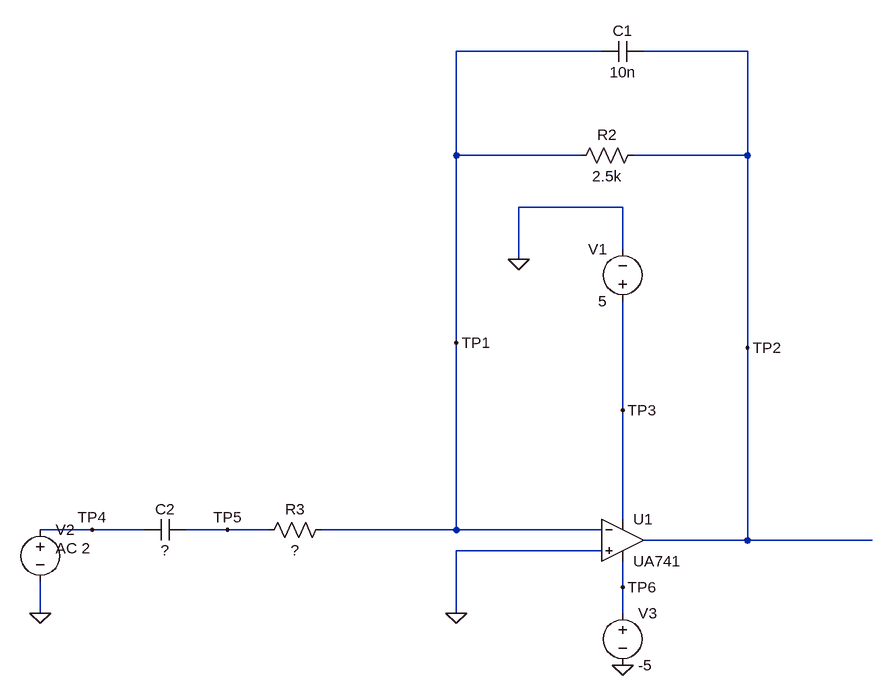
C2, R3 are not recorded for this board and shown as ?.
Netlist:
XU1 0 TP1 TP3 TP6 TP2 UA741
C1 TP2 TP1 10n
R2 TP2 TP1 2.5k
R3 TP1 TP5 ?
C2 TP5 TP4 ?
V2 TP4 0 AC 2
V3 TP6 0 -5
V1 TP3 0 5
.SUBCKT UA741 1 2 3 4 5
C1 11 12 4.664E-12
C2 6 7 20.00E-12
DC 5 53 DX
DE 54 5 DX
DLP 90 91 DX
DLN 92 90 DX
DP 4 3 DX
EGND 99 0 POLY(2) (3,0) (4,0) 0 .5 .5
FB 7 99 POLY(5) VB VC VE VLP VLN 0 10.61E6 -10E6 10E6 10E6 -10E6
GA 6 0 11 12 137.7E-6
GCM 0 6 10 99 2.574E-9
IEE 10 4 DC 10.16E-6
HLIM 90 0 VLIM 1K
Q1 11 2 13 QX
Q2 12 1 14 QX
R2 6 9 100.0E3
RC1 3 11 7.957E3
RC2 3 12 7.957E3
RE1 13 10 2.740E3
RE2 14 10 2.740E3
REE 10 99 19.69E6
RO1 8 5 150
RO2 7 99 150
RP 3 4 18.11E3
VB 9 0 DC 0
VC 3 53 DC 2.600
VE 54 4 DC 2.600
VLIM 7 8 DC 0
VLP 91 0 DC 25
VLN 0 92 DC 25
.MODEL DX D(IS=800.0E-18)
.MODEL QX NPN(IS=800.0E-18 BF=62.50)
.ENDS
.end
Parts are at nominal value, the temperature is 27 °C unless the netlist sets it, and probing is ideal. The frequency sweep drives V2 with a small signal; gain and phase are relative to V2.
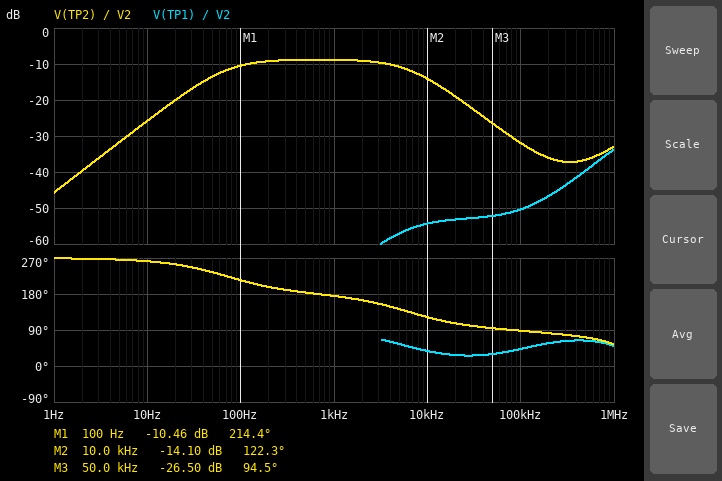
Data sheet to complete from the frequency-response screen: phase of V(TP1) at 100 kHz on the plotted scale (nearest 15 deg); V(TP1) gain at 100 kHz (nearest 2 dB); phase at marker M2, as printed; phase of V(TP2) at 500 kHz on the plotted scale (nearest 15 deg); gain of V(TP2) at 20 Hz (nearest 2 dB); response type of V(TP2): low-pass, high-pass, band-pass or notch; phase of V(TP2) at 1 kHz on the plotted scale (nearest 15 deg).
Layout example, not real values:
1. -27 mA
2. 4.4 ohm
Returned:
1. 45 deg
2. -50 dB
3. 122.3 deg
4. 75 deg
5. -20 dB
6. band-pass
7. 180 deg
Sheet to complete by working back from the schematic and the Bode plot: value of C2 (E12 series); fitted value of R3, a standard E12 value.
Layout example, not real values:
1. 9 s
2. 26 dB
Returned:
1. 330 nF
2. 6.8 kΩ
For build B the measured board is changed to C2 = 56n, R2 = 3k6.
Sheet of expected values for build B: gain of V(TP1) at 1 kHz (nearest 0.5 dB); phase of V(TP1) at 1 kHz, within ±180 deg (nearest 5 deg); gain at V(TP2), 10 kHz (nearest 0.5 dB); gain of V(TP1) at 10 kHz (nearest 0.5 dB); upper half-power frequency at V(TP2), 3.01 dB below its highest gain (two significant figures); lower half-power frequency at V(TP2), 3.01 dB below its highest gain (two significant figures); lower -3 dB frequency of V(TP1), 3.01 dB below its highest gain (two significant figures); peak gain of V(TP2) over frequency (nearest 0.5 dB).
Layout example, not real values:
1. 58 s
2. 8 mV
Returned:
1. -67.0 dB
2. 100 deg
3. -13.5 dB
4. -54.0 dB
5. 5.2 kHz
6. 360 Hz
7. 940 kHz
8. -6.5 dB
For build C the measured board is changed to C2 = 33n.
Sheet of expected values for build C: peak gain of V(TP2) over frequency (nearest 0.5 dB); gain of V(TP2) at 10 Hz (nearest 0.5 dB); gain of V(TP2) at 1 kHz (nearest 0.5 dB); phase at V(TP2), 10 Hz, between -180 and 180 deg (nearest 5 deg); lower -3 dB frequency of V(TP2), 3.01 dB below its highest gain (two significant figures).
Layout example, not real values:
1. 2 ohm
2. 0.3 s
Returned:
1. -9.5 dB
2. -45.5 dB
3. -10.5 dB
4. -90 deg
5. 590 Hz
